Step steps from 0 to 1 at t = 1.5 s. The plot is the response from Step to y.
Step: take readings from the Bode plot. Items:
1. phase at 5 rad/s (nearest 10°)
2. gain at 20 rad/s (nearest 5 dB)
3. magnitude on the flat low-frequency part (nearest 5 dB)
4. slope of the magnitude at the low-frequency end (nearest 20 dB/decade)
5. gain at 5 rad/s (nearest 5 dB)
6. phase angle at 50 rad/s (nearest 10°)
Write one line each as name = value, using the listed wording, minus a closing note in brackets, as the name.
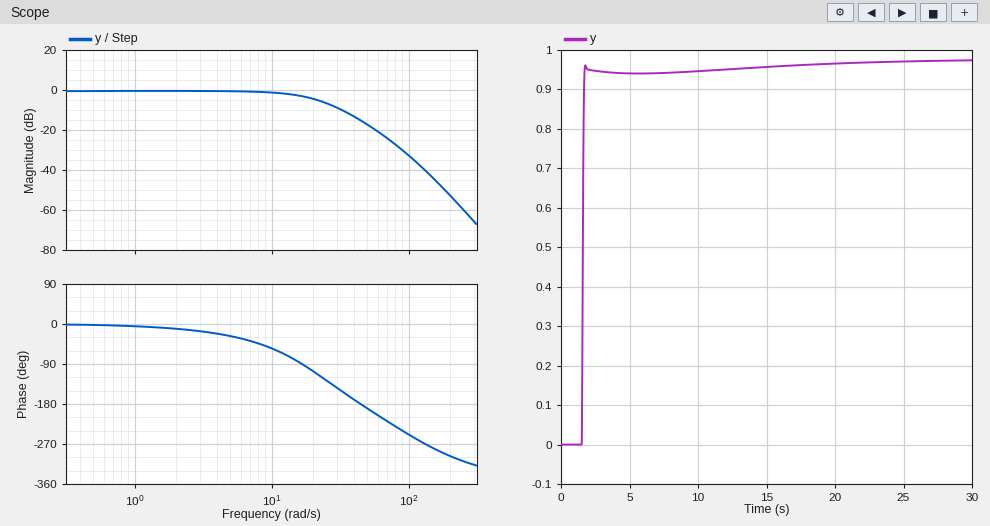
phase at 5 rad/s = -30°
gain at 20 rad/s = -5 dB
magnitude on the flat low-frequency part = 0 dB
slope of the magnitude at the low-frequency end = 0 dB/decade
gain at 5 rad/s = 0 dB
phase angle at 50 rad/s = -190°
